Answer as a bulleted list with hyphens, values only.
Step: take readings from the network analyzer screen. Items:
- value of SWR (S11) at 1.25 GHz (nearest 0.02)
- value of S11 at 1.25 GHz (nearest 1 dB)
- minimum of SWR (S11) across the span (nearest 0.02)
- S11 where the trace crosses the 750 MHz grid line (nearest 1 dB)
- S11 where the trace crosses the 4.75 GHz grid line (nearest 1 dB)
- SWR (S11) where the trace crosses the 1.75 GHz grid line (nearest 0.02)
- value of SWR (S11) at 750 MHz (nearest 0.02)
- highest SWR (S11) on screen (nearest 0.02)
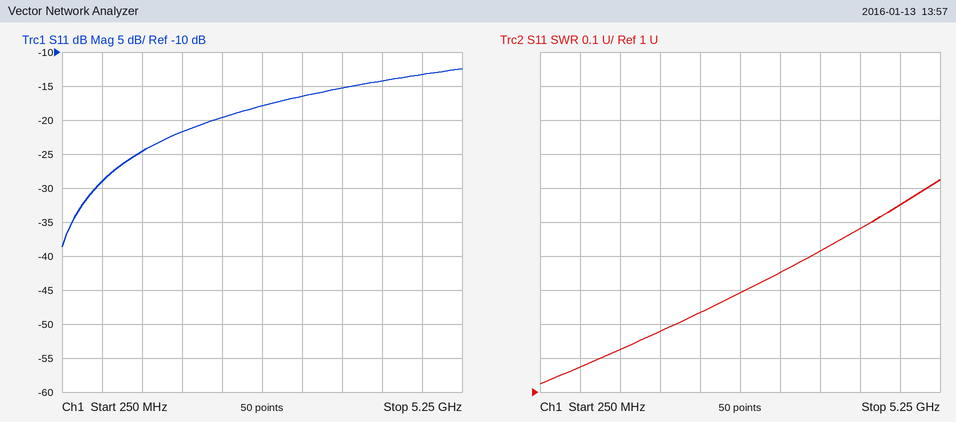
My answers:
- 1.12
- -25 dB
- 1.02
- -29 dB
- -13 dB
- 1.18
- 1.08
- 1.62
